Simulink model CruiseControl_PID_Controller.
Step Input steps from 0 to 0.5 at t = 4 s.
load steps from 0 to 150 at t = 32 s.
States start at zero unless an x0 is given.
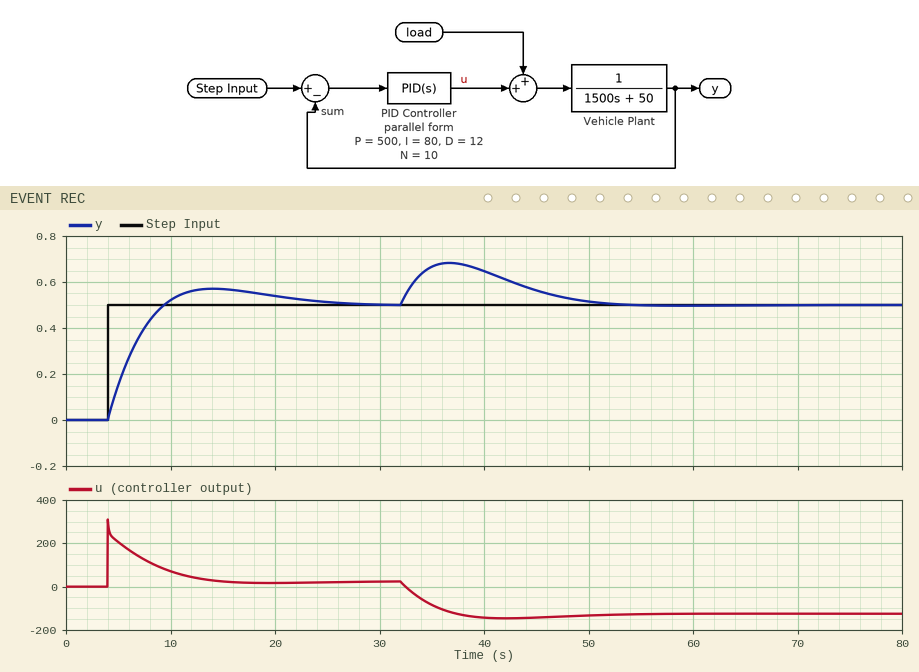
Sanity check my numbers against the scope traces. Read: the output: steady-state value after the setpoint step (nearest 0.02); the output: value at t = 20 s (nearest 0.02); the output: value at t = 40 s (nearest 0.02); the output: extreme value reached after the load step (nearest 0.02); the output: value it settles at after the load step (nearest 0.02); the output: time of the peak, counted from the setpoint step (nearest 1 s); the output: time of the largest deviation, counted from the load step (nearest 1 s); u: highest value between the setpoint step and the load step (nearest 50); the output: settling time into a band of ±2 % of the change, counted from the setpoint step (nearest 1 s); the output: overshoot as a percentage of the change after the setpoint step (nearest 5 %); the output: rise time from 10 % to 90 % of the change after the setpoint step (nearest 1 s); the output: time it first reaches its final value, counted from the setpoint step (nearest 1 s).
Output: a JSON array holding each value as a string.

["0.50", "0.54", "0.64", "0.68", "0.50", "10 s", "5 s", "300", "22 s", "15 %", "4 s", "5 s"]
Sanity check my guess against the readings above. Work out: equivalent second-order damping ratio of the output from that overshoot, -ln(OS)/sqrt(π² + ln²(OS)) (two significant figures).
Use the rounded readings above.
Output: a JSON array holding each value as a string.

["0.52"]
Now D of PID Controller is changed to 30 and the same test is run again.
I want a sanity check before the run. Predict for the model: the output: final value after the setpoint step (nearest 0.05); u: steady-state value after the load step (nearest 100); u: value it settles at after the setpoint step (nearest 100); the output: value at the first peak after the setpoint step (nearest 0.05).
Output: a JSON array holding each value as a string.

["0.50", "-100", "0", "0.55"]
